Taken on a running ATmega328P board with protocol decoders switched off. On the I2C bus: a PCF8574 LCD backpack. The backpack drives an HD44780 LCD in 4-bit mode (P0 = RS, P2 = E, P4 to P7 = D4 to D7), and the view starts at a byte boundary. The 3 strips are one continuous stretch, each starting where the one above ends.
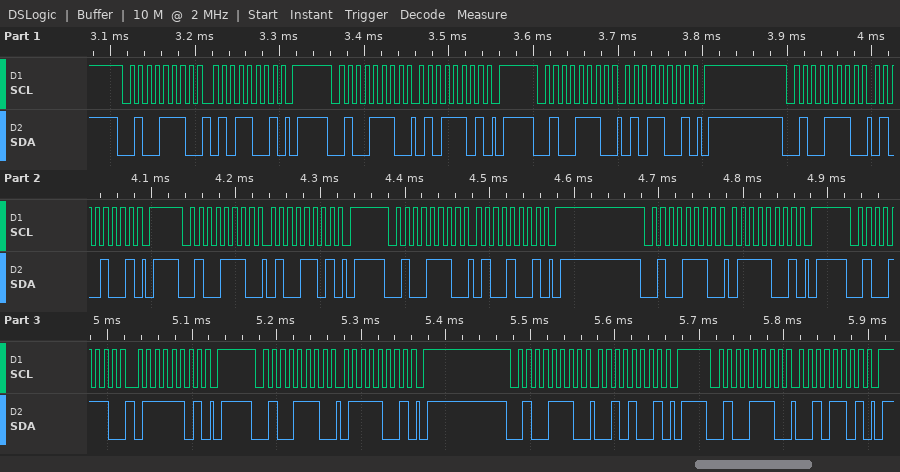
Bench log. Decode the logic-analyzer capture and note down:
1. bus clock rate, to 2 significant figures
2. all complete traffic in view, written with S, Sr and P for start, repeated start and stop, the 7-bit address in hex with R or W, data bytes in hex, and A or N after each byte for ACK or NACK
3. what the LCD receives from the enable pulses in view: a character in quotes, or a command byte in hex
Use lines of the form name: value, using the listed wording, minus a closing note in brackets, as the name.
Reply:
bus clock rate, to 2 significant figures: 100 kHz
all complete traffic in view, written with S, Sr and P for start, repeated start and stop, the 7-bit address in hex with R or W, data bytes in hex, and A or N after each byte for ACK or NACK: S 27W A 59 A P S 27W A 5D A P S 27W A 59 A P S 27W A 49 A P S 27W A 4D A P S 27W A 49 A P S 27W A 79 A P S 27W A 7D A P S 27W A 79 A P S 27W A 29 A P S 27W A 2D A P
what the LCD receives from the enable pulses in view: a character in quotes, or a command byte in hex: 'T'
